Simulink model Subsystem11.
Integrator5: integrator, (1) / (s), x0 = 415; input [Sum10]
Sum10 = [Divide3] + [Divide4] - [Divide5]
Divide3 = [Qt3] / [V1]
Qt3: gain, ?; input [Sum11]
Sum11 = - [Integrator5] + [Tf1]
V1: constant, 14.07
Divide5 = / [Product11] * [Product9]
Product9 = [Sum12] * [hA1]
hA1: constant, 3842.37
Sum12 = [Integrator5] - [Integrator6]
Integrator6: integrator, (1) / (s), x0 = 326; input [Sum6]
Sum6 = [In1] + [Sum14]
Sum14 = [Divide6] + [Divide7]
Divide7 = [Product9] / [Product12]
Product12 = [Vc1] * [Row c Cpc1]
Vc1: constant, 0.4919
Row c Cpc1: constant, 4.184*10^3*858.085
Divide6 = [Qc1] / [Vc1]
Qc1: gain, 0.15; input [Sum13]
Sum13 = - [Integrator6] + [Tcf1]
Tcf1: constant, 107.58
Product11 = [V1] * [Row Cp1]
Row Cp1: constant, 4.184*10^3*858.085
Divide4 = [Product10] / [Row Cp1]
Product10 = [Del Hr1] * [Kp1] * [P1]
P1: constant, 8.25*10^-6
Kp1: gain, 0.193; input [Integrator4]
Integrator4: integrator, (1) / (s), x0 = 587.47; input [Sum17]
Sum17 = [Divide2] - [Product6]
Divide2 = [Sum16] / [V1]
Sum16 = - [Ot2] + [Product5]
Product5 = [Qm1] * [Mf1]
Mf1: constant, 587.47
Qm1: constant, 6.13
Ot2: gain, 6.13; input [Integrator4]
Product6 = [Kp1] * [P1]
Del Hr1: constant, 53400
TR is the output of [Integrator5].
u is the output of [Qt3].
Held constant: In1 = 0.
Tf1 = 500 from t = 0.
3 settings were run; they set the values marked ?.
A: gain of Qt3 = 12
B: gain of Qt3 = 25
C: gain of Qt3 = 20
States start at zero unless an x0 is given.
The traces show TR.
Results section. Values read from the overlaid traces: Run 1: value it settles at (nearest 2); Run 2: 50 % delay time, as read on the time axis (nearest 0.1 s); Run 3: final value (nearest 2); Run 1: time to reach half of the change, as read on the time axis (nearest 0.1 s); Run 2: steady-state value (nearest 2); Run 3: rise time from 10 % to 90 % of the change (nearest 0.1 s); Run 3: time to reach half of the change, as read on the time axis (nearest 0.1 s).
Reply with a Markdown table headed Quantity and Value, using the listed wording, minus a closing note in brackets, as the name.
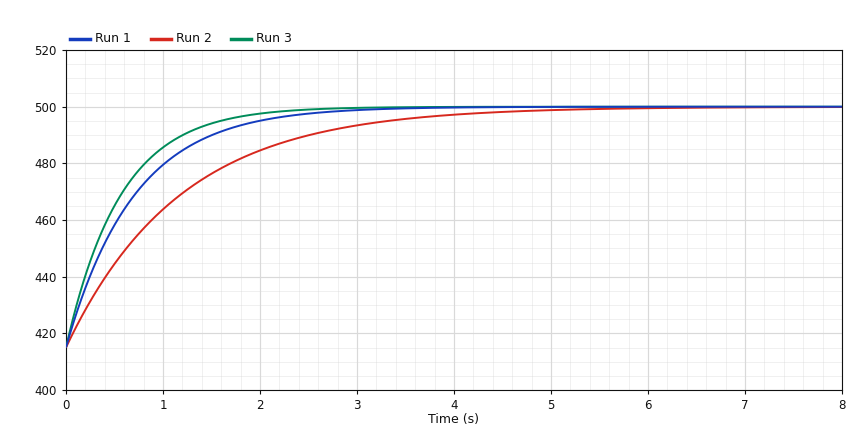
| Quantity | Value |
|---|---|
| Run 1: value it settles at | 500 |
| Run 2: 50 % delay time, as read on the time axis | 0.8 s |
| Run 3: final value | 500 |
| Run 1: time to reach half of the change, as read on the time axis | 0.5 s |
| Run 2: steady-state value | 500 |
| Run 3: rise time from 10 % to 90 % of the change | 1.2 s |
| Run 3: time to reach half of the change, as read on the time axis | 0.4 s |
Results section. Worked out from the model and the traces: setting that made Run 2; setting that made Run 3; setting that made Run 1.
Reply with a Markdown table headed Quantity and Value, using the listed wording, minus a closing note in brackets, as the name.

| Quantity | Value |
|---|---|
| setting that made Run 2 | A |
| setting that made Run 3 | B |
| setting that made Run 1 | C |
